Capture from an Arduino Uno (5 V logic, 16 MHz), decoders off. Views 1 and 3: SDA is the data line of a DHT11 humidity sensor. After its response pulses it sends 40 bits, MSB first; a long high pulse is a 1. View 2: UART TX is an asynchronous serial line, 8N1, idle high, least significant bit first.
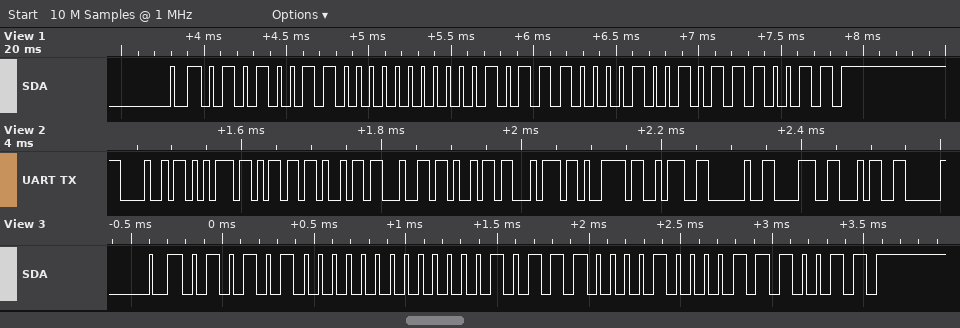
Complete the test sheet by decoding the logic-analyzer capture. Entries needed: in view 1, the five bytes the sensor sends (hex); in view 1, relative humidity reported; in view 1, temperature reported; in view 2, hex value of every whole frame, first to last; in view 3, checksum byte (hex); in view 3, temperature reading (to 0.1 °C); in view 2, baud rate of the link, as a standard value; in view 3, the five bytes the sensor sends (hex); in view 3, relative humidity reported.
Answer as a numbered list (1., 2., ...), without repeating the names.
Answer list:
1. 53 00 17 09 73
2. 83 %
3. 23.9 °C
4. 48 75 6D 69 64 69 74 79 3A 20 38 34
5. 0x73
6. 23.8 °C
7. 115200 baud
8. 54 00 17 08 73
9. 84 %
